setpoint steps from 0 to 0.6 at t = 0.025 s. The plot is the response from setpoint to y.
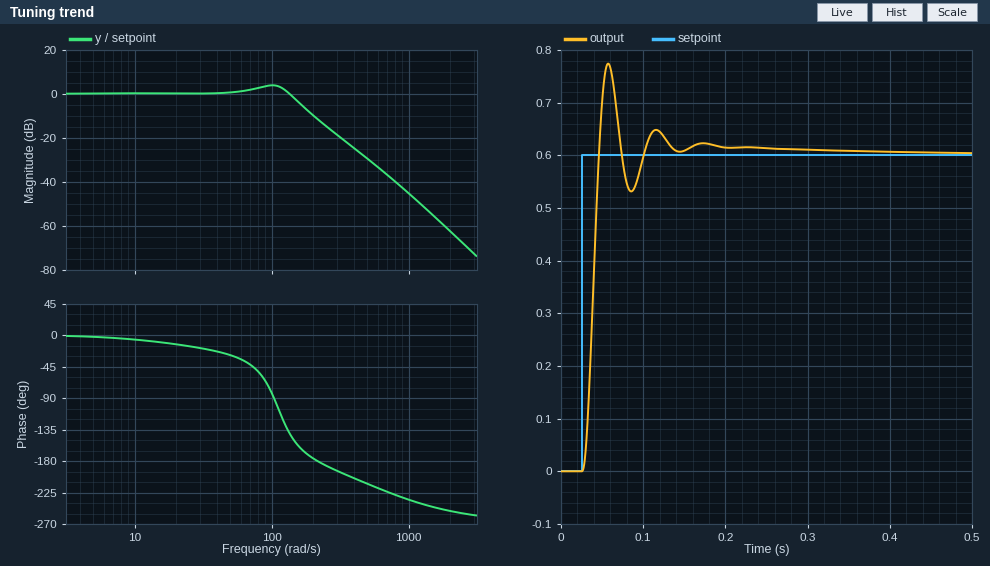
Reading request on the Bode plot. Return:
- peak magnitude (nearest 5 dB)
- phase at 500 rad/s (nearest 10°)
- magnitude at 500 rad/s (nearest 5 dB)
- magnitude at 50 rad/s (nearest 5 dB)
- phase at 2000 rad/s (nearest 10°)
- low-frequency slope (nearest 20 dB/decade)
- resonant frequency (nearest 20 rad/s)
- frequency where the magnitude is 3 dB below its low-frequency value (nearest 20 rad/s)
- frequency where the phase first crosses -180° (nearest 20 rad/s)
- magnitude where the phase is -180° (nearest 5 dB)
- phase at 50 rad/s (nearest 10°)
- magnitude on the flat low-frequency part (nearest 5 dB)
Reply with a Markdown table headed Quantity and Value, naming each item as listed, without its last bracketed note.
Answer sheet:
| Quantity | Value |
|---|---|
| peak magnitude | 5 dB |
| phase at 500 rad/s | -210° |
| magnitude at 500 rad/s | -30 dB |
| magnitude at 50 rad/s | 0 dB |
| phase at 2000 rad/s | -250° |
| low-frequency slope | 0 dB/decade |
| resonant frequency | 100 rad/s |
| frequency where the magnitude is 3 dB below its low-frequency value | 160 rad/s |
| frequency where the phase first crosses -180° | 220 rad/s |
| magnitude where the phase is -180° | -10 dB |
| phase at 50 rad/s | -30° |
| magnitude on the flat low-frequency part | 0 dB |
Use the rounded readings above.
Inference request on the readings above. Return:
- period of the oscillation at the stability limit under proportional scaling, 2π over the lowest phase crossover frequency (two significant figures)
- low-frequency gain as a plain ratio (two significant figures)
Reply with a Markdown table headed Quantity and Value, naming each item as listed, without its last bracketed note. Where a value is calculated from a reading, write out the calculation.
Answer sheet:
| Quantity | Value |
|---|---|
| period of the oscillation at the stability limit under proportional scaling, 2π over the lowest phase crossover frequency | 2π / 220 = 0.029 s |
| low-frequency gain as a plain ratio | 10^(0 / 20) = 1.0 |
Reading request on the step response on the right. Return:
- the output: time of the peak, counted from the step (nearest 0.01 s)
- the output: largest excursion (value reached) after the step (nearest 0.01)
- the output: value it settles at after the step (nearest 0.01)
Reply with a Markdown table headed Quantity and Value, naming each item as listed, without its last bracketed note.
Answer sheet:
| Quantity | Value |
|---|---|
| the output: time of the peak, counted from the step | 0.03 s |
| the output: largest excursion (value reached) after the step | 0.77 |
| the output: value it settles at after the step | 0.60 |
